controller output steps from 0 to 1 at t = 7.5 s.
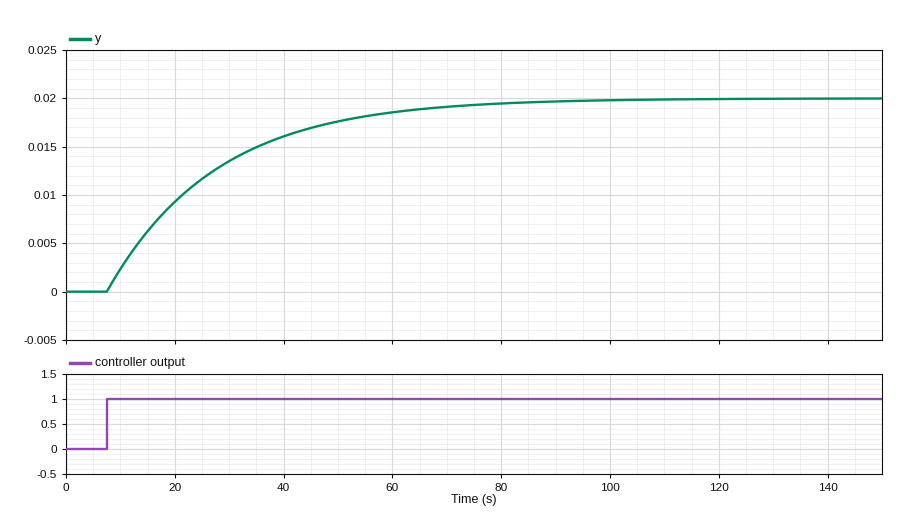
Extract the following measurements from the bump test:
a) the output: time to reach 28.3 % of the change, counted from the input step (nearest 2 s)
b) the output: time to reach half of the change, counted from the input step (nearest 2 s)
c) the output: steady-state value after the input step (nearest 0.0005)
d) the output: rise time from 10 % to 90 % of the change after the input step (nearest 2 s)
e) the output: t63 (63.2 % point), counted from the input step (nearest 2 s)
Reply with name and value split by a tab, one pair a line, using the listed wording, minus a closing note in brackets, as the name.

the output: time to reach 28.3 % of the change, counted from the input step	6 s
the output: time to reach half of the change, counted from the input step	14 s
the output: steady-state value after the input step	0.0200
the output: rise time from 10 % to 90 % of the change after the input step	44 s
the output: t63 (63.2 % point), counted from the input step	20 s
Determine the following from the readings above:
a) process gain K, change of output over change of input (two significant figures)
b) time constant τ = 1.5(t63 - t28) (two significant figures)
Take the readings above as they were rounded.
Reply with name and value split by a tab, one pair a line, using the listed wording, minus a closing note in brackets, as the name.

process gain K, change of output over change of input	0.020
time constant τ = 1.5(t63 - t28)	21 s
